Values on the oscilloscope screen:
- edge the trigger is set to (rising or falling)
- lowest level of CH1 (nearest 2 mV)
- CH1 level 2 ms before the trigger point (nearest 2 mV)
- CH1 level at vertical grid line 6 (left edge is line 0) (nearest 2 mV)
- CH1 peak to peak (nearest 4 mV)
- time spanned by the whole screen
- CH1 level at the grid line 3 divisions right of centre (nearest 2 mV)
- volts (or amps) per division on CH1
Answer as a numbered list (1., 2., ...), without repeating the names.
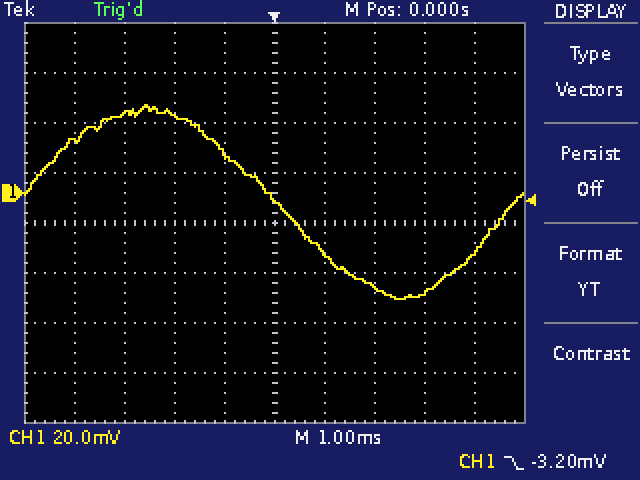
1. falling
2. -42 mV
3. 30 mV
4. -24 mV
5. 76 mV
6. 10 ms
7. -40 mV
8. 20 mV
